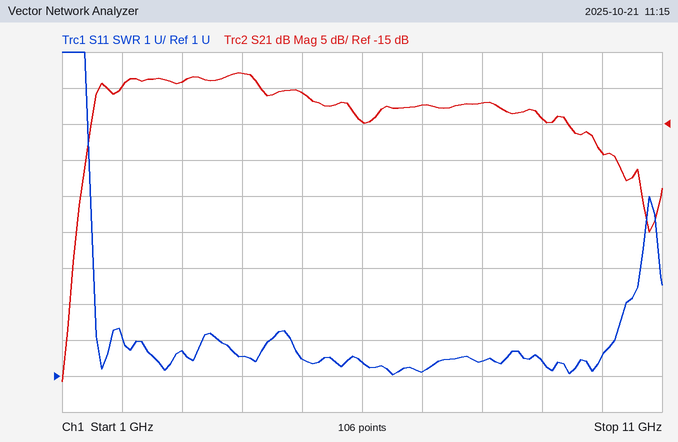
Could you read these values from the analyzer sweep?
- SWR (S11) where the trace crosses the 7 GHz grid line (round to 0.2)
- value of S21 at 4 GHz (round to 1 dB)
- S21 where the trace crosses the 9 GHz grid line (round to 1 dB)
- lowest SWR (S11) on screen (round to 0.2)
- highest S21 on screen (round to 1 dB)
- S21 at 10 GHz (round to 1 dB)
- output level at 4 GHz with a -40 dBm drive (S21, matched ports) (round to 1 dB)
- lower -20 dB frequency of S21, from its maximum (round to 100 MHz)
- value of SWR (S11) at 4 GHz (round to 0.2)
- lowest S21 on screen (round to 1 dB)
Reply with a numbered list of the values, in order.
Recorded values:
1. 1.2
2. -8 dB
3. -14 dB
4. 1.0
5. -8 dB
6. -19 dB
7. -48 dBm
8. 1.3 GHz
9. 1.6
10. -51 dB
